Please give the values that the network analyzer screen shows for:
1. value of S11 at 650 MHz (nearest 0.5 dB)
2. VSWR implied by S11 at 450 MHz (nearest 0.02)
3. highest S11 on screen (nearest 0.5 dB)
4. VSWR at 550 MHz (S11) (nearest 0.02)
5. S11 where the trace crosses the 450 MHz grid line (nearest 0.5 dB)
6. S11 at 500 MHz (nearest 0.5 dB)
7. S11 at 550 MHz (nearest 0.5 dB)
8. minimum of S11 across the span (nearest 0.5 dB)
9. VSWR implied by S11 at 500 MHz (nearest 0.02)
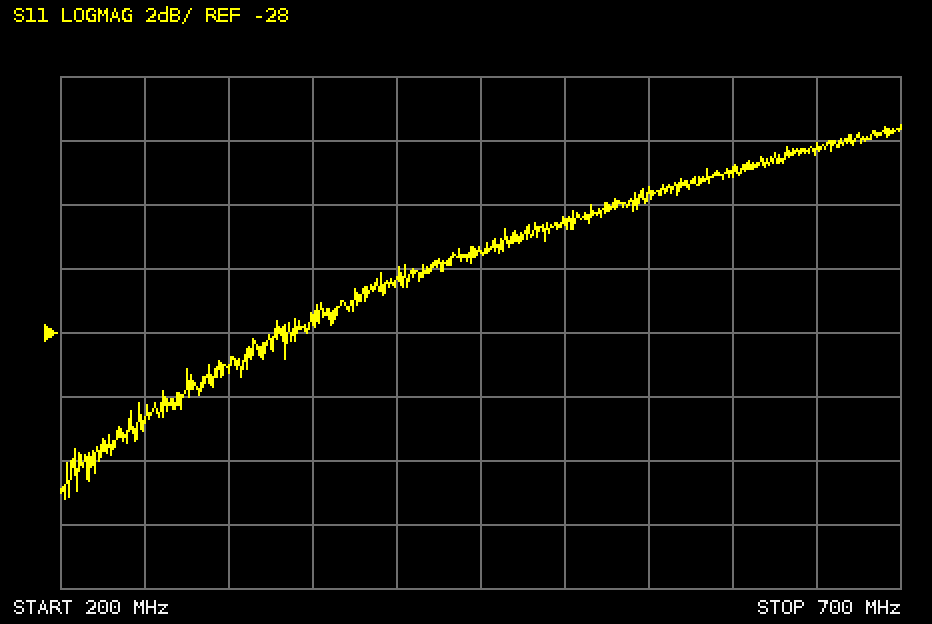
-22.0 dB
1.12
-21.5 dB
1.14
-25.5 dB
-24.5 dB
-23.5 dB
-33.0 dB
1.12
